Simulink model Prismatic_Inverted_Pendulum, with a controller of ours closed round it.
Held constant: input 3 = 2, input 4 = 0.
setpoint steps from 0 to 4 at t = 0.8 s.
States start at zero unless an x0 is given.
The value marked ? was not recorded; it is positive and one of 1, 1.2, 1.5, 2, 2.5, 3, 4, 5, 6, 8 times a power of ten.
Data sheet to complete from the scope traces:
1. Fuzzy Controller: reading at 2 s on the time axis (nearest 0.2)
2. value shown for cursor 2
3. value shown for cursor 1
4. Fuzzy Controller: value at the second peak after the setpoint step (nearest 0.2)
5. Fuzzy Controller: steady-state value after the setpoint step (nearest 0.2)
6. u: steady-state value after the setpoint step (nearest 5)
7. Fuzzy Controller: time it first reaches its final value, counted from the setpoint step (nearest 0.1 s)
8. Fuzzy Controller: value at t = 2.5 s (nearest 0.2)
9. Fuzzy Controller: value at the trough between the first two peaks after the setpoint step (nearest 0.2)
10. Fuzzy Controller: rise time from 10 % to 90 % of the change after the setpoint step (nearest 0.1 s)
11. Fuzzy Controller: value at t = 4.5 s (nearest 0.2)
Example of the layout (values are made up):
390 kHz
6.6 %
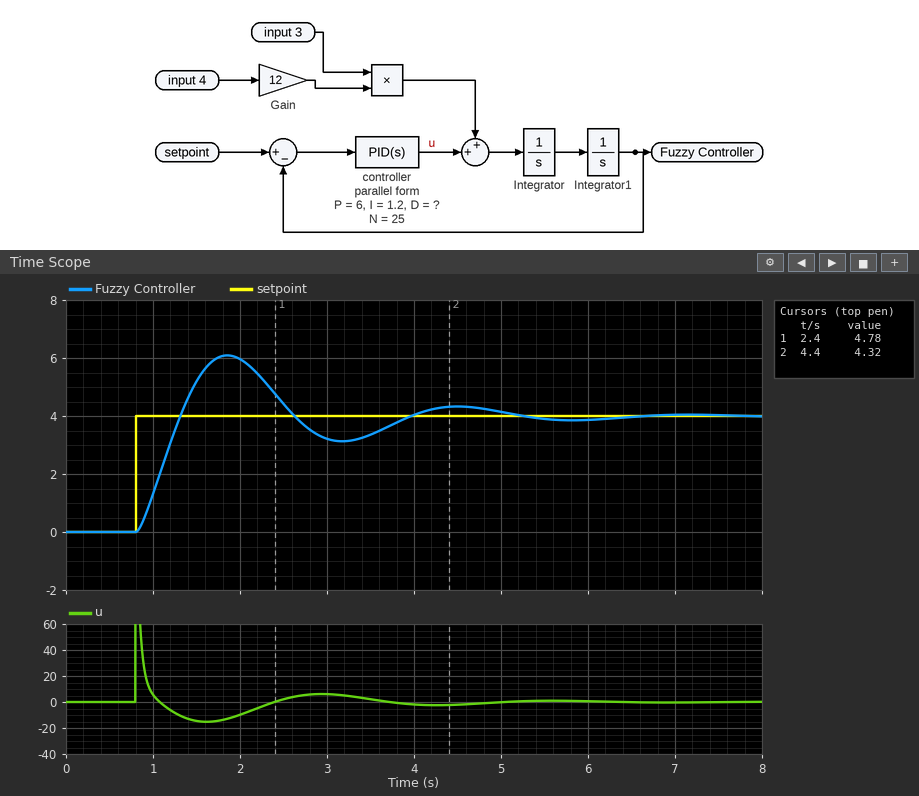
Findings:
6.0
4.32
4.78
4.4
4.0
0
0.5 s
4.4
3.2
0.4 s
4.4
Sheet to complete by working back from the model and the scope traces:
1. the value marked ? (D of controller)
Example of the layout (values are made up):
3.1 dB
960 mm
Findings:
1.5
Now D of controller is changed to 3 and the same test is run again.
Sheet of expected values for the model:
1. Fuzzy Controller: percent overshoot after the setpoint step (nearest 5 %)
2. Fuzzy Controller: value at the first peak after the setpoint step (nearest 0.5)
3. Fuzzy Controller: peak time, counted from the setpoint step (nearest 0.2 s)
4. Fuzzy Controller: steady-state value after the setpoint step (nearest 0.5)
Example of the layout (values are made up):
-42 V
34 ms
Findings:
30 %
5.0
0.8 s
4.0
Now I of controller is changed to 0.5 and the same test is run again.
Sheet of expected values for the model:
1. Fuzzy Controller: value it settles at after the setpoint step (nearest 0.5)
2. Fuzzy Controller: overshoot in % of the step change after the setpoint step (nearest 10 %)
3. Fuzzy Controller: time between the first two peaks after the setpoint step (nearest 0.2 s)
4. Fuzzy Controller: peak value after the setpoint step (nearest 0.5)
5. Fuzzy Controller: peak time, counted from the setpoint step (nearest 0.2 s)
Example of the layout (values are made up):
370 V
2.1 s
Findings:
4.0
50 %
2.6 s
6.0
1.0 s
